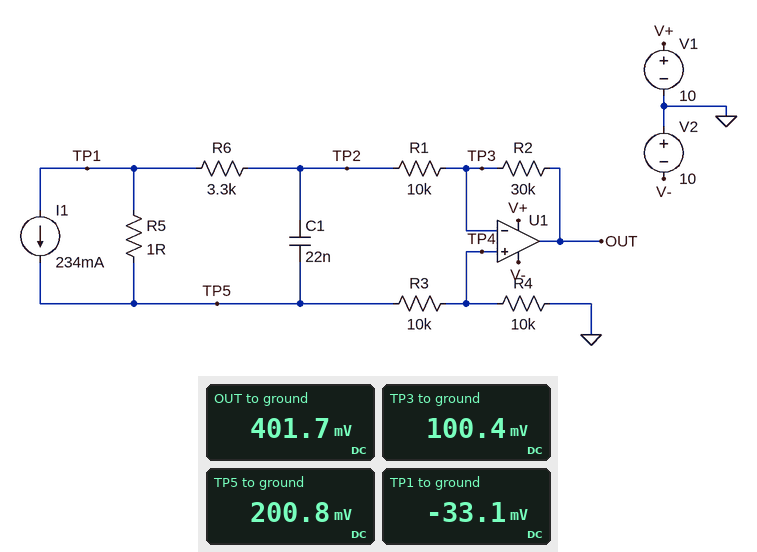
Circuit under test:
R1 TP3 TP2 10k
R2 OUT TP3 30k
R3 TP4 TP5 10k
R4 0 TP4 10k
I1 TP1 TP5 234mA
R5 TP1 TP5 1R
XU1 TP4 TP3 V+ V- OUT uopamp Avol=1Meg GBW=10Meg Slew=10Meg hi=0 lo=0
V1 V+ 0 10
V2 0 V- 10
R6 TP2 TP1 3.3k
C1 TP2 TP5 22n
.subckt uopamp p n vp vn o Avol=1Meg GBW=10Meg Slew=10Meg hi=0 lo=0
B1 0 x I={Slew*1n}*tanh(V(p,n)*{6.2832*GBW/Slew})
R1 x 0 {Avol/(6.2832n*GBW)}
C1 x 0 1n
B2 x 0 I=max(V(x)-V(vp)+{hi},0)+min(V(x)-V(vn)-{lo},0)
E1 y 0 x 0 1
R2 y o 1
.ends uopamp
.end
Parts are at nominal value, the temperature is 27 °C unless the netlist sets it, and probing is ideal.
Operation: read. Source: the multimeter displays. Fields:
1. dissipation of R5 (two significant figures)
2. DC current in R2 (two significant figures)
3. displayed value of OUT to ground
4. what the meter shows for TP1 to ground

55 mW
10 µA
401.7 mV
-33.1 mV
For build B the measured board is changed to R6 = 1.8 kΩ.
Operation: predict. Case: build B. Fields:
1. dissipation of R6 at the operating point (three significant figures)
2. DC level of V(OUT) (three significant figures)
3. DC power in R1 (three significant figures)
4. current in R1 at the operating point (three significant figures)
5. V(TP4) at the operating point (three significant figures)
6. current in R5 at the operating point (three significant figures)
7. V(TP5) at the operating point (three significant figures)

207 nW
429 mV
1.15 µW
10.7 µA
107 mV
234 mA
215 mV
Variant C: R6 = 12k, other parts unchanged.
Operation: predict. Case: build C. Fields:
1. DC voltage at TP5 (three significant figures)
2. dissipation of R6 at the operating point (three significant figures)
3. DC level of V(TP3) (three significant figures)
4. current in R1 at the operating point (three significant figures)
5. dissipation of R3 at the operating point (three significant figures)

146 mV
642 nW
73.1 mV
7.31 µA
535 nW
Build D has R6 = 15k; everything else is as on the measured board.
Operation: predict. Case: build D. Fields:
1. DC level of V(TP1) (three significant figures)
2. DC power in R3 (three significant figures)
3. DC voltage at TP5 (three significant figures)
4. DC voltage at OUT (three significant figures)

-100 mV
447 nW
134 mV
267 mV
